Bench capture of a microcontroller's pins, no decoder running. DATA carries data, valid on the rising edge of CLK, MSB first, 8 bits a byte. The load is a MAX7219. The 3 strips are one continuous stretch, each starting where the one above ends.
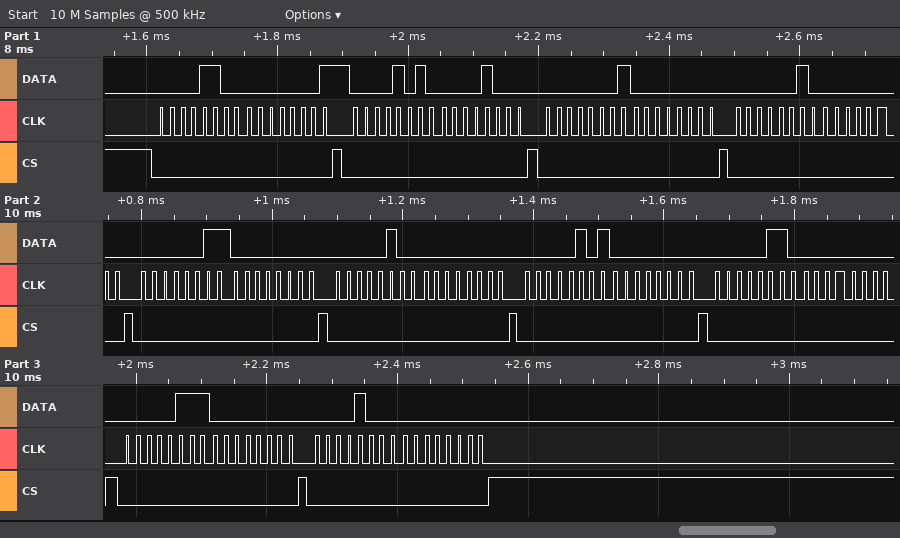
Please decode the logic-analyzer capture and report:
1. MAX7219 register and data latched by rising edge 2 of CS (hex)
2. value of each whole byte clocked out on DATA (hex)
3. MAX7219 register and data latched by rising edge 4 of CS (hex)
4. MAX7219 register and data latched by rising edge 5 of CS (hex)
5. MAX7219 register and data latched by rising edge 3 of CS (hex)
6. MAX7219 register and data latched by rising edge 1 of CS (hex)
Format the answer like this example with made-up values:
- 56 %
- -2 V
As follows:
- register 0xA, data 0x08
- 0x0C 0x01 0x0A 0x08 0x01 0x00 0x02 0x00 0x03 0x00 0x04 0x00 0x05 0x00 0x06 0x00 0x07 0x00 0x08 0x00
- register 0x2, data 0x00
- register 0x3, data 0x00
- register 0x1, data 0x00
- register 0xC, data 0x01
